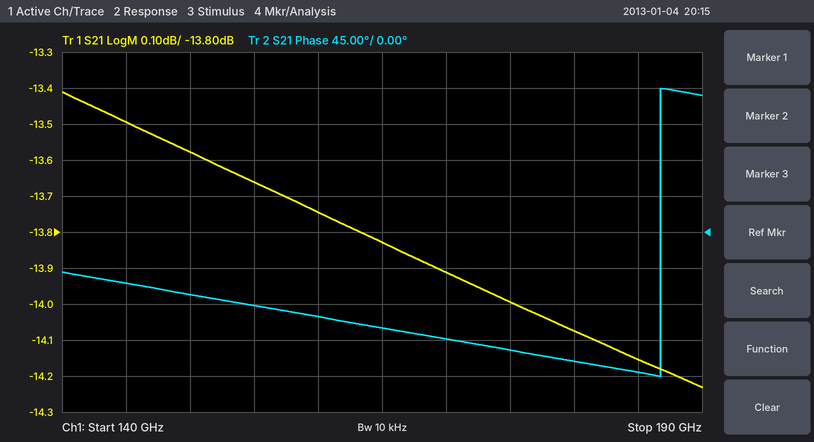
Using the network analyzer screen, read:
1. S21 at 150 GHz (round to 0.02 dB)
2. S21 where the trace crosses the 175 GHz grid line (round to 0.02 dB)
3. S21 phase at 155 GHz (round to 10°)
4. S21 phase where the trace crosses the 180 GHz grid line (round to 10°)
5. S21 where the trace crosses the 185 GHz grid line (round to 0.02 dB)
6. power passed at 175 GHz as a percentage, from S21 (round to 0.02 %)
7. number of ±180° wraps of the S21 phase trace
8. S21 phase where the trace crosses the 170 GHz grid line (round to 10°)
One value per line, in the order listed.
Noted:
-13.58 dB
-14.00 dB
-90°
-160°
-14.16 dB
3.98 %
1
-130°
